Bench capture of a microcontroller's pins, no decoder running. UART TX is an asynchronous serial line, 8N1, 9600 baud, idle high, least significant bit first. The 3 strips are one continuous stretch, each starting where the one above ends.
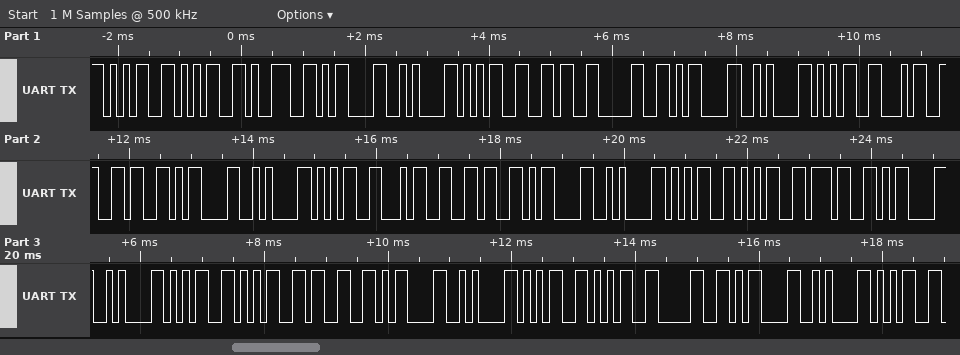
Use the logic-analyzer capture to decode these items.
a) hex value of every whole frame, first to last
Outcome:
35 35 39 0D 0A 35 36 30 0D 0A 35 34 36 0D 0A 35 34 36 0D 0A 35 35 37 0D 0A 35 35 33 0D 0A 35 35 30 0D 0A 35
